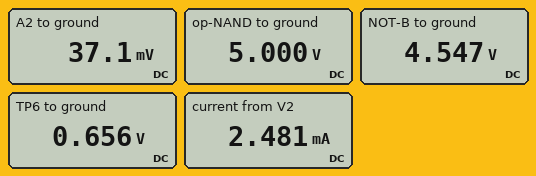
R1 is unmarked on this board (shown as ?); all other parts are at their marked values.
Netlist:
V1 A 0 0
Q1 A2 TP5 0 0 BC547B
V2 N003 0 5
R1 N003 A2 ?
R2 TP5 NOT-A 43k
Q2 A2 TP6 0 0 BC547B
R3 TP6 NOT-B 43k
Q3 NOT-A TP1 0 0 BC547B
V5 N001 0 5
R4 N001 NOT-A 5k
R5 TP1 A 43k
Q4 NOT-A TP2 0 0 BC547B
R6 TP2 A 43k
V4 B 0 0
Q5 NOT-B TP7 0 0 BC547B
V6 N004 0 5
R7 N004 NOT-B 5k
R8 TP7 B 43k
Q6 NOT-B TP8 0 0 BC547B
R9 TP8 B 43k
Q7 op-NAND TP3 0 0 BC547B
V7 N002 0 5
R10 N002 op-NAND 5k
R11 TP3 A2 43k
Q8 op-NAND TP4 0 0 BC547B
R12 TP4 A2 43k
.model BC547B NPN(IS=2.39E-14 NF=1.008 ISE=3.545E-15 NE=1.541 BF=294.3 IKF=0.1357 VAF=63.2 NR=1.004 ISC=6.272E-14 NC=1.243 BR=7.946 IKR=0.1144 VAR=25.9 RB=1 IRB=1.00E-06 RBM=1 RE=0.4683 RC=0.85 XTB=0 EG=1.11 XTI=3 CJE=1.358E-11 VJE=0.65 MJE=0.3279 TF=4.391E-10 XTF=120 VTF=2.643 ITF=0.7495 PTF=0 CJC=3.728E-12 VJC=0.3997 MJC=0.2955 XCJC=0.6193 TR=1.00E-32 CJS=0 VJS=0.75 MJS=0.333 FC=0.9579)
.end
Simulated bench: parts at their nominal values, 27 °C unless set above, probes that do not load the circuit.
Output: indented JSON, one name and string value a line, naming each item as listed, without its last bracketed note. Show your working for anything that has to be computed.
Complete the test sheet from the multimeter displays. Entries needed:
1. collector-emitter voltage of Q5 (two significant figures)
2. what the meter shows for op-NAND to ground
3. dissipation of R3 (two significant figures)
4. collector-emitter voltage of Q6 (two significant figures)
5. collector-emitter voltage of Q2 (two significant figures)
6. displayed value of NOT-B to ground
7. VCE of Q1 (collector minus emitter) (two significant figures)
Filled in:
{
  "collector-emitter voltage of Q5": "4.547 V = 4.5 V",
  "what the meter shows for op-NAND to ground": "5.000 V",
  "dissipation of R3": "(4.547 V - 656 mV)^2 / 43 kΩ = 350 µW",
  "collector-emitter voltage of Q6": "4.547 V = 4.5 V",
  "collector-emitter voltage of Q2": "37.1 mV = 37 mV",
  "displayed value of NOT-B to ground": "4.547 V",
  "VCE of Q1 (collector minus emitter)": "37.1 mV = 37 mV"
}
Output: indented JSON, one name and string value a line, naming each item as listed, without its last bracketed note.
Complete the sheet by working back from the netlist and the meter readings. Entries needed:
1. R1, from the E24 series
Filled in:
{
  "R1, from the E24 series": "2 kΩ"
}
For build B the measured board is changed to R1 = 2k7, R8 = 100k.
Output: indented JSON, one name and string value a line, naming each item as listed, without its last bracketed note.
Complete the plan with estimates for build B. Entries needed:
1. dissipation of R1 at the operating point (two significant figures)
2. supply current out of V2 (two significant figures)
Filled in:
{
  "dissipation of R1 at the operating point": "9.1 mW",
  "supply current out of V2": "1.8 mA"
}
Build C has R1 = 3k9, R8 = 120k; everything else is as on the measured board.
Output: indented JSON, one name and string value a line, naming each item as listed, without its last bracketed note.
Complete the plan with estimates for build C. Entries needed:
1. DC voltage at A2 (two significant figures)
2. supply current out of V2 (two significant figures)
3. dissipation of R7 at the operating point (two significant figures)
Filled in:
{
  "DC voltage at A2": "26 mV",
  "supply current out of V2": "1.3 mA",
  "dissipation of R7 at the operating point": "41 µW"
}
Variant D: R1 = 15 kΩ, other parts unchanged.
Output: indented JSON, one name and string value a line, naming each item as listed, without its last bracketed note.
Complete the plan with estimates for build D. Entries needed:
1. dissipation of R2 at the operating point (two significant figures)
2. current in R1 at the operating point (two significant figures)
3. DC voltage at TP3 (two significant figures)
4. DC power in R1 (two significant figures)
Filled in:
{
  "dissipation of R2 at the operating point": "360 µW",
  "current in R1 at the operating point": "330 µA",
  "DC voltage at TP3": "13 mV",
  "DC power in R1": "1.7 mW"
}
